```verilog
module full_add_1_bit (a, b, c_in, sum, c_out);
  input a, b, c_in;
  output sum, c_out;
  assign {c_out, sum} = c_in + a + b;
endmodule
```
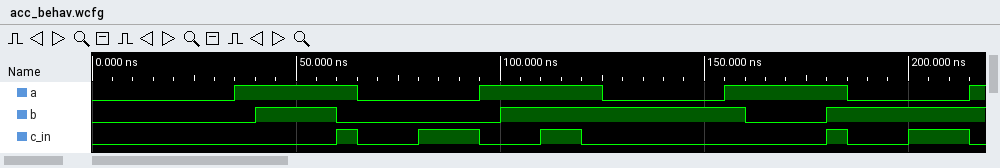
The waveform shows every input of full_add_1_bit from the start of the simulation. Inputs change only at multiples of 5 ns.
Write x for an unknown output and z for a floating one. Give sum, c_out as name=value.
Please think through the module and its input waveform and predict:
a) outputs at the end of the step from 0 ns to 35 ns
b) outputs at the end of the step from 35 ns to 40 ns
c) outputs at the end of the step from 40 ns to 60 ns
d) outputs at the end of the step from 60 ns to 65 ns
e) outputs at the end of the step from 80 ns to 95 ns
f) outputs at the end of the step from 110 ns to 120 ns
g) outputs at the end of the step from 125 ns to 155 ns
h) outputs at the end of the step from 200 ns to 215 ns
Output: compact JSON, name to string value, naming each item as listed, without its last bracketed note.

{"outputs at the end of the step from 0 ns to 35 ns": "sum=0, c_out=0", "outputs at the end of the step from 35 ns to 40 ns": "sum=1, c_out=0", "outputs at the end of the step from 40 ns to 60 ns": "sum=0, c_out=1", "outputs at the end of the step from 60 ns to 65 ns": "sum=0, c_out=1", "outputs at the end of the step from 80 ns to 95 ns": "sum=1, c_out=0", "outputs at the end of the step from 110 ns to 120 ns": "sum=1, c_out=1", "outputs at the end of the step from 125 ns to 155 ns": "sum=1, c_out=0", "outputs at the end of the step from 200 ns to 215 ns": "sum=0, c_out=1"}
